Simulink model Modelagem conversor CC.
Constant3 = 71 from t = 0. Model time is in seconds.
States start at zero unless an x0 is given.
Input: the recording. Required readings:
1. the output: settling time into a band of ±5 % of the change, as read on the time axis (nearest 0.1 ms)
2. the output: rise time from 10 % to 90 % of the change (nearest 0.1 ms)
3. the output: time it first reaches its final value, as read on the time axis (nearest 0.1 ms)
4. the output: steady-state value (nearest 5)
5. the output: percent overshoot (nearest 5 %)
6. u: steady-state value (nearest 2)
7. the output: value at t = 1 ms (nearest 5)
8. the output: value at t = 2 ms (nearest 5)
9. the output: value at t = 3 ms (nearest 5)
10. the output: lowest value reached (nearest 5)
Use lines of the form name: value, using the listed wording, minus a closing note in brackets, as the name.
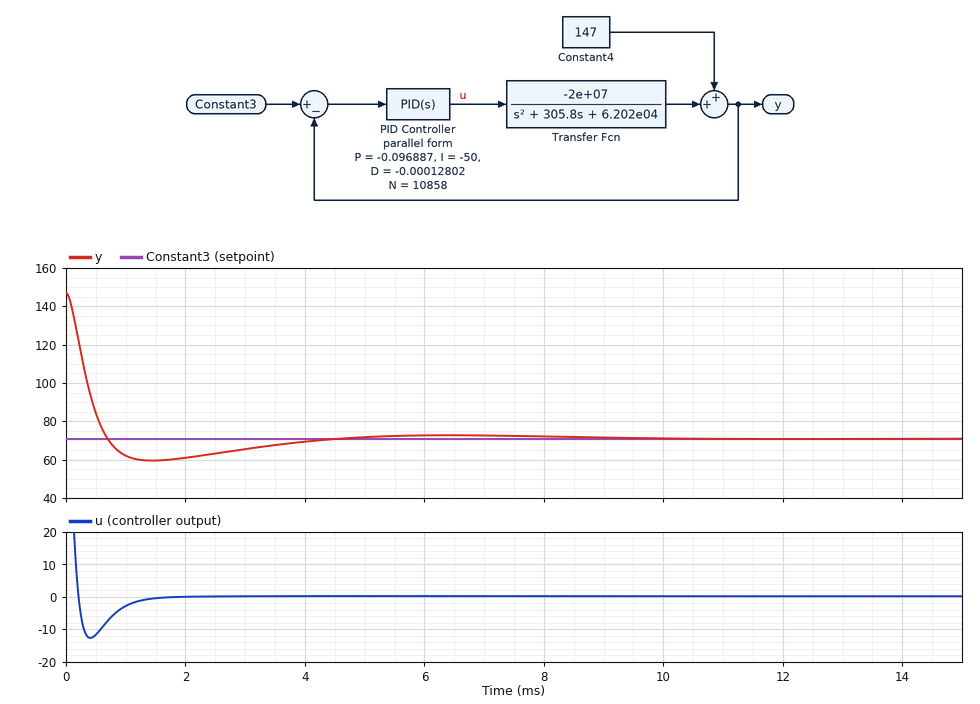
the output: settling time into a band of ±5 % of the change, as read on the time axis: 3.4 ms
the output: rise time from 10 % to 90 % of the change: 0.5 ms
the output: time it first reaches its final value, as read on the time axis: 0.7 ms
the output: steady-state value: 70
the output: percent overshoot: 15 %
u: steady-state value: 0
the output: value at t = 1 ms: 60
the output: value at t = 2 ms: 60
the output: value at t = 3 ms: 65
the output: lowest value reached: 60
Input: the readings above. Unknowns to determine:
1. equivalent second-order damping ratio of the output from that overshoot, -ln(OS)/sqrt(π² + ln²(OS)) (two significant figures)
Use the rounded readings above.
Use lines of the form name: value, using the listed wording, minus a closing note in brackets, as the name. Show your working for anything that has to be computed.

equivalent second-order damping ratio of the output from that overshoot, -ln(OS)/sqrt(π² + ln²(OS)): ln(0.15) = -1.897; 1.897 / sqrt(9.870 + 3.599) = 0.52
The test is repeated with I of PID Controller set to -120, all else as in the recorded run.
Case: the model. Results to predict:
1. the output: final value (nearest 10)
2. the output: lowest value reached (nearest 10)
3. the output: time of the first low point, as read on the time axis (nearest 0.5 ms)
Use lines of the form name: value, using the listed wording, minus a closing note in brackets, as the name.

the output: final value: 70
the output: lowest value reached: 50
the output: time of the first low point, as read on the time axis: 1.5 ms
